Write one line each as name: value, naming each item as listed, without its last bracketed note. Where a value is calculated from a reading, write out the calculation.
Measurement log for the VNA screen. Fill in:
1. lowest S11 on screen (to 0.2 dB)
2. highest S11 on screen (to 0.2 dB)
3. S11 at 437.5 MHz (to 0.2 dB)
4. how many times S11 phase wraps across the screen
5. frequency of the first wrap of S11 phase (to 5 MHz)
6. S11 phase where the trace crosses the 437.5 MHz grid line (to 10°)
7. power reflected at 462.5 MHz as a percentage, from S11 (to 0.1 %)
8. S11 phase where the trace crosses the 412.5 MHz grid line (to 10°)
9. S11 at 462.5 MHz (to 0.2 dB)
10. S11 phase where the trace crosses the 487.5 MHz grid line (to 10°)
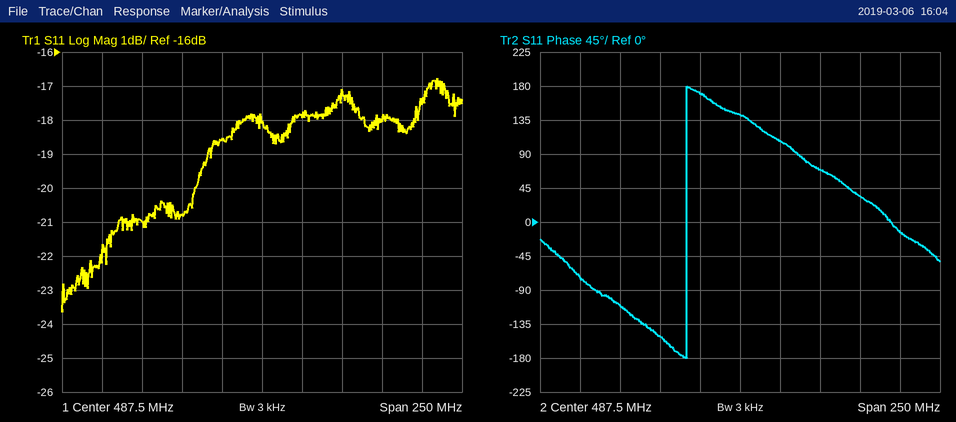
lowest S11 on screen: -23.6 dB
highest S11 on screen: -16.8 dB
S11 at 437.5 MHz: -20.8 dB
how many times S11 phase wraps across the screen: 1
frequency of the first wrap of S11 phase: 455 MHz
S11 phase where the trace crosses the 437.5 MHz grid line: -150°
power reflected at 462.5 MHz as a percentage, from S11: 10^(-18.6/10) ≈ 1.4 %
S11 phase where the trace crosses the 412.5 MHz grid line: -110°
S11 at 462.5 MHz: -18.6 dB
S11 phase where the trace crosses the 487.5 MHz grid line: 140°
